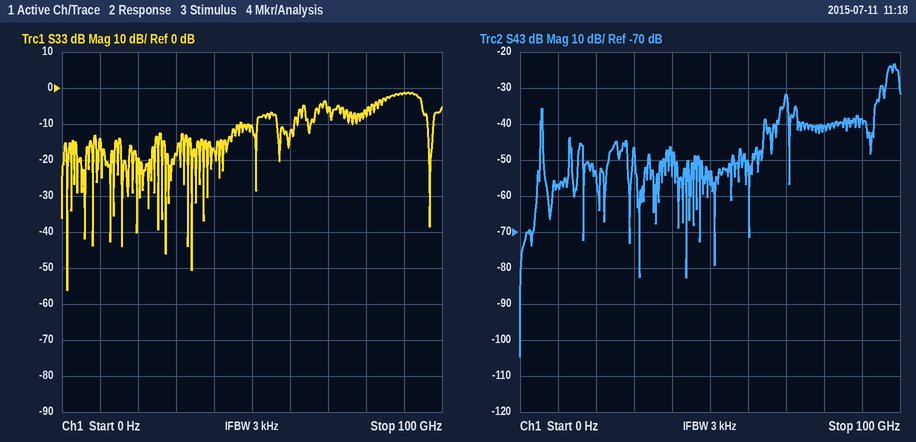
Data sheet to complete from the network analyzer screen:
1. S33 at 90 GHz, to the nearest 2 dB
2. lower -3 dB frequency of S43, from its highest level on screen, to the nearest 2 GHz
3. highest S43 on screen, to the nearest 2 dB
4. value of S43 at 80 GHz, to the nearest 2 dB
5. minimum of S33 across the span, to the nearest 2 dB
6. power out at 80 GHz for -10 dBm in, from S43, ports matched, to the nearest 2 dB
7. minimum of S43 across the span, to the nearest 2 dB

-2 dB
96 GHz
-24 dB
-40 dB
-56 dB
-50 dBm
-104 dB
